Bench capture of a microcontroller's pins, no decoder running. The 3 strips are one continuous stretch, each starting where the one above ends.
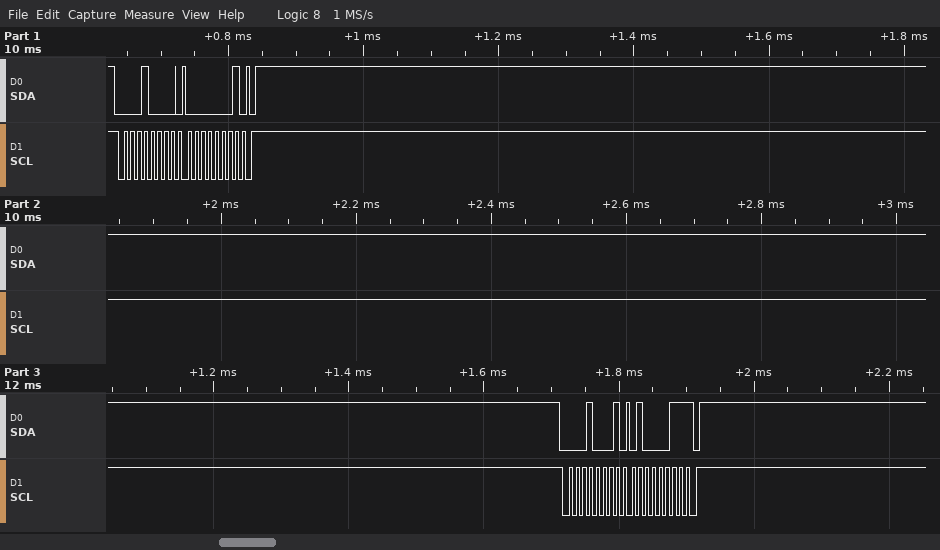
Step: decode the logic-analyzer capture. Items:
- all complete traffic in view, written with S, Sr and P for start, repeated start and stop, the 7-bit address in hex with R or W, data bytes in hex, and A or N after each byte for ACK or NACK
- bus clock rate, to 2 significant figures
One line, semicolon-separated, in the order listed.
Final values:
S 08W A 01 A P S 08R A 43 N P; 100 kHz
